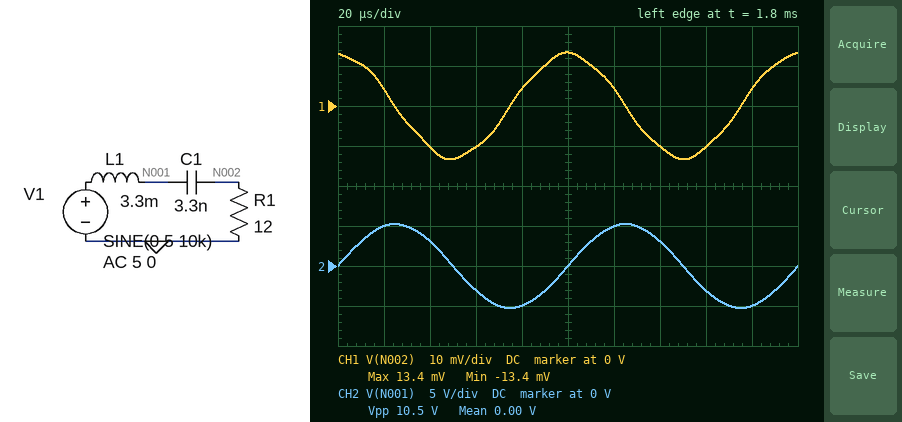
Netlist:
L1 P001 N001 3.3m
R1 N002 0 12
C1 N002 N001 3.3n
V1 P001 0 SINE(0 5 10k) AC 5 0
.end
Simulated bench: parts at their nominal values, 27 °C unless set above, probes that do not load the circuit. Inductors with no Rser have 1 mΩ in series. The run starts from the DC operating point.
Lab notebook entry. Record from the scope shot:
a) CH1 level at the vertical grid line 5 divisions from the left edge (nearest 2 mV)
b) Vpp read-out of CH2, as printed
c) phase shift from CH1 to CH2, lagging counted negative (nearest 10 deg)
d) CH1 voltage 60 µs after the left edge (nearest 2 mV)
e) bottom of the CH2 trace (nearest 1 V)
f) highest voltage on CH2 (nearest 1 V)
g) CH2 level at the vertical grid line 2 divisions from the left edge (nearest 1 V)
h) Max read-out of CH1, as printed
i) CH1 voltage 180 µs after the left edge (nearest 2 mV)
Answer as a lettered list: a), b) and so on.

a) 14 mV
b) 10.5 V
c) -90 deg
d) -10 mV
e) -5 V
f) 5 V
g) 3 V
h) 13.4 mV
i) 4 mV
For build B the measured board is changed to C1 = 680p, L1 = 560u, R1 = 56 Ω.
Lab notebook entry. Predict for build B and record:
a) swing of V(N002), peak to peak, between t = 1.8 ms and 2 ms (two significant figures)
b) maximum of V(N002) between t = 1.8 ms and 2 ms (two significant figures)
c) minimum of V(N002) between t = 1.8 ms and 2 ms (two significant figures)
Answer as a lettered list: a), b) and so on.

a) 24 mV
b) 12 mV
c) -12 mV
